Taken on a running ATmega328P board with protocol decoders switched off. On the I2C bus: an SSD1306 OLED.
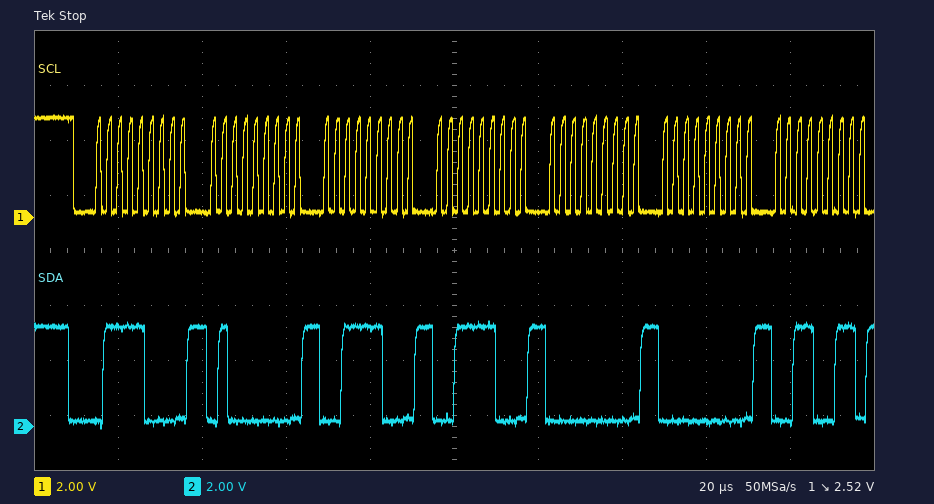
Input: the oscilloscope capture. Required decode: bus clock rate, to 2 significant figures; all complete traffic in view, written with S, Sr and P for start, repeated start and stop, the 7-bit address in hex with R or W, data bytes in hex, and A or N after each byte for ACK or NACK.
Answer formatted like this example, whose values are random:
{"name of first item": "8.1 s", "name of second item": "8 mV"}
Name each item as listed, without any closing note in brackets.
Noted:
{"bus clock rate, to 2 significant figures": "400 kHz", "all complete traffic in view, written with S, Sr and P for start, repeated start and stop, the 7-bit address in hex with R or W, data bytes in hex, and A or N after each byte for ACK or NACK": "S 3CW A 40 A 3C A 3C A 00 A 00 A 33 A"}
